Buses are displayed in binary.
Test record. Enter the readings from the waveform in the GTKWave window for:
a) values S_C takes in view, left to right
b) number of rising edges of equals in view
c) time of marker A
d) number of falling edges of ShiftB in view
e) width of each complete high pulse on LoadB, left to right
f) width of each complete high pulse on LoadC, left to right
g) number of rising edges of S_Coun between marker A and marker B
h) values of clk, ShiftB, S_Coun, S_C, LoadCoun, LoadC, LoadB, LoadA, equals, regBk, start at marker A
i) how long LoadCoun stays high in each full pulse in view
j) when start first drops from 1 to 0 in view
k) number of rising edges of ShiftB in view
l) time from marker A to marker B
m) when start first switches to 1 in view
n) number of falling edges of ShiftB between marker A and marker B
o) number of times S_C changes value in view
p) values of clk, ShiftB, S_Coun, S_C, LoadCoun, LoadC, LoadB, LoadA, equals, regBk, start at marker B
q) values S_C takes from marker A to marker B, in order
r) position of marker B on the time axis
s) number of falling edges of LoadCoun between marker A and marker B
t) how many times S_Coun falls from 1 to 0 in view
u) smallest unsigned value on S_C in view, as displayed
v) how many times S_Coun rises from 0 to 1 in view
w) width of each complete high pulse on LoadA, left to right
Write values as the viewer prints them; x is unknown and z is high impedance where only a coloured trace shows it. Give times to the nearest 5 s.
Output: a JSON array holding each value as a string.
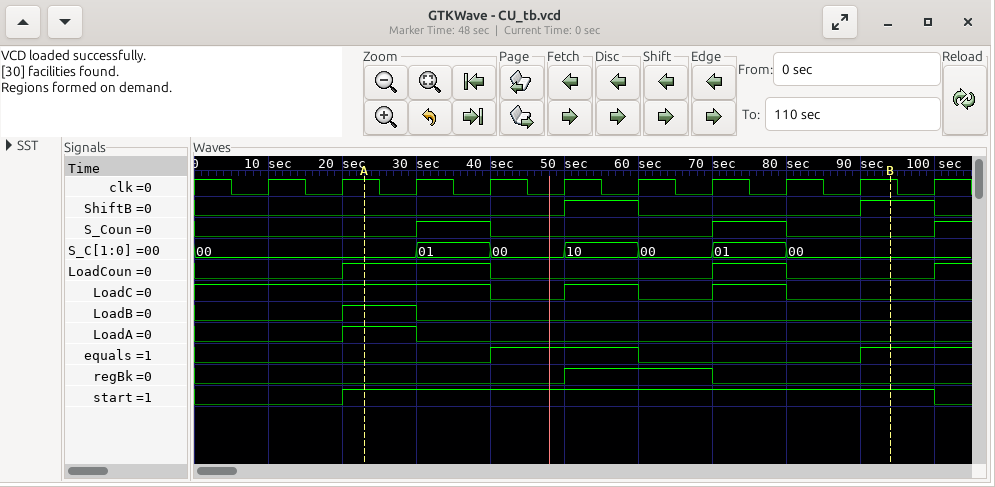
["00, 01, 00, 10, 00, 01, 00", "2", "25 s", "2", "10 s", "10 s, 10 s", "2", "clk=1, ShiftB=0, S_Coun=0, S_C=00, LoadCoun=1, LoadC=1, LoadB=1, LoadA=1, equals=0, regBk=0, start=1", "20 s, 10 s", "100 s", "2", "70 s", "20 s", "1", "6", "clk=1, ShiftB=1, S_Coun=0, S_C=00, LoadCoun=0, LoadC=0, LoadB=0, LoadA=0, equals=1, regBk=0, start=1", "00, 01, 00, 10, 00, 01, 00", "95 s", "2", "2", "00", "3", "10 s"]
